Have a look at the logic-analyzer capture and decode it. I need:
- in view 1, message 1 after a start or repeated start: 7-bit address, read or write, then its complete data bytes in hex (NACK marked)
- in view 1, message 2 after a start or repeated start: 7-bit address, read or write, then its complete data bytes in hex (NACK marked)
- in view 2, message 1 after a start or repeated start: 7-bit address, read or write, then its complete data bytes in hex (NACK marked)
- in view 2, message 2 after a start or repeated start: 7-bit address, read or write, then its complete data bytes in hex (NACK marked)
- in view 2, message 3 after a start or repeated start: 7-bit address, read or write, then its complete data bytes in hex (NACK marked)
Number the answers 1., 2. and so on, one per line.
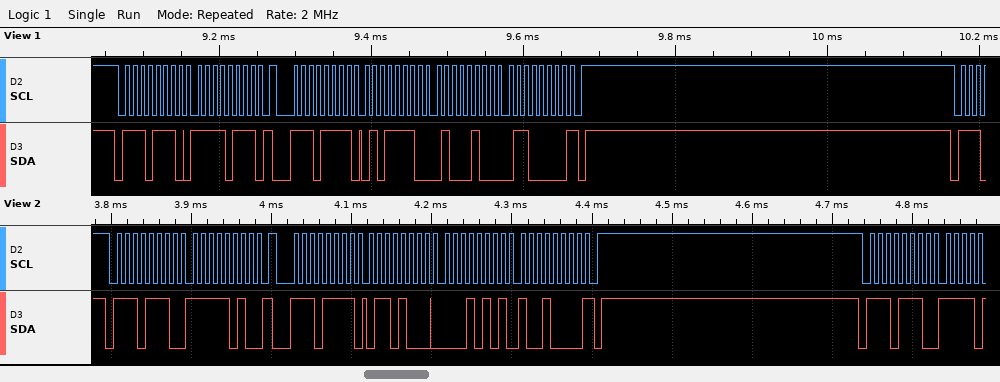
1. 0x77 write: F7
2. 0x77 read: 5E 44 60 NACK
3. 0x77 write: FA
4. 0x77 read: 68 15 90 NACK
5. 0x77 write
